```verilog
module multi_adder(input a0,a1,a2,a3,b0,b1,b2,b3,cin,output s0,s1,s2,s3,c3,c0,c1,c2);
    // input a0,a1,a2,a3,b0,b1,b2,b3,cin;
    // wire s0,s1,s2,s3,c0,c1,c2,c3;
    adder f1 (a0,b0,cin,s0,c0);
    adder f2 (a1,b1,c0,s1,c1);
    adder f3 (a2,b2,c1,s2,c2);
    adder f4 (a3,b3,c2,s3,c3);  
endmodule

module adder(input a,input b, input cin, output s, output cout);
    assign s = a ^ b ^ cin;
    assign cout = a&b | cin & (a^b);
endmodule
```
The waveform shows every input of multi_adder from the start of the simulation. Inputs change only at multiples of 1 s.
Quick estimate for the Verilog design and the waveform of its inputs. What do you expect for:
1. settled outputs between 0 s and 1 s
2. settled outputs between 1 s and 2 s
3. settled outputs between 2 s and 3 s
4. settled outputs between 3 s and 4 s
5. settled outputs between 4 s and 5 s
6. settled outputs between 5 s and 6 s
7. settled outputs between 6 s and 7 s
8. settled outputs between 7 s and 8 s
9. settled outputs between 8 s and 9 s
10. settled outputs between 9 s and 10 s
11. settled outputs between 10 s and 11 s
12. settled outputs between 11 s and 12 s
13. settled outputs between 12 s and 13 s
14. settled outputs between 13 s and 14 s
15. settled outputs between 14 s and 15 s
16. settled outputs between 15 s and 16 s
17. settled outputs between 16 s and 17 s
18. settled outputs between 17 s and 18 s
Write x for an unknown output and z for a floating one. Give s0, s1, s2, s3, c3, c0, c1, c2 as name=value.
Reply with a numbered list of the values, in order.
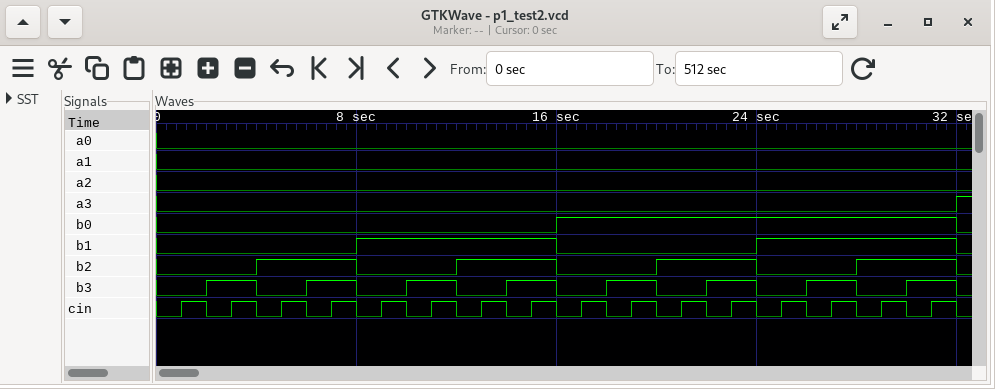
1. s0=0, s1=0, s2=0, s3=0, c3=0, c0=0, c1=0, c2=0
2. s0=1, s1=0, s2=0, s3=0, c3=0, c0=0, c1=0, c2=0
3. s0=0, s1=0, s2=0, s3=1, c3=0, c0=0, c1=0, c2=0
4. s0=1, s1=0, s2=0, s3=1, c3=0, c0=0, c1=0, c2=0
5. s0=0, s1=0, s2=1, s3=0, c3=0, c0=0, c1=0, c2=0
6. s0=1, s1=0, s2=1, s3=0, c3=0, c0=0, c1=0, c2=0
7. s0=0, s1=0, s2=1, s3=1, c3=0, c0=0, c1=0, c2=0
8. s0=1, s1=0, s2=1, s3=1, c3=0, c0=0, c1=0, c2=0
9. s0=0, s1=1, s2=0, s3=0, c3=0, c0=0, c1=0, c2=0
10. s0=1, s1=1, s2=0, s3=0, c3=0, c0=0, c1=0, c2=0
11. s0=0, s1=1, s2=0, s3=1, c3=0, c0=0, c1=0, c2=0
12. s0=1, s1=1, s2=0, s3=1, c3=0, c0=0, c1=0, c2=0
13. s0=0, s1=1, s2=1, s3=0, c3=0, c0=0, c1=0, c2=0
14. s0=1, s1=1, s2=1, s3=0, c3=0, c0=0, c1=0, c2=0
15. s0=0, s1=1, s2=1, s3=1, c3=0, c0=0, c1=0, c2=0
16. s0=1, s1=1, s2=1, s3=1, c3=0, c0=0, c1=0, c2=0
17. s0=1, s1=0, s2=0, s3=0, c3=0, c0=0, c1=0, c2=0
18. s0=0, s1=1, s2=0, s3=0, c3=0, c0=1, c1=0, c2=0
